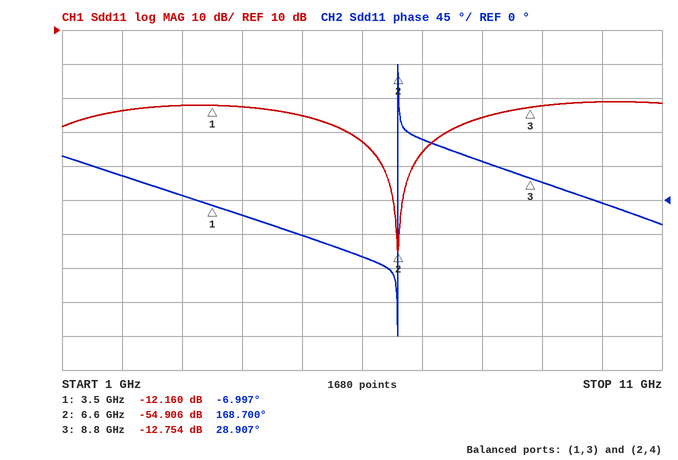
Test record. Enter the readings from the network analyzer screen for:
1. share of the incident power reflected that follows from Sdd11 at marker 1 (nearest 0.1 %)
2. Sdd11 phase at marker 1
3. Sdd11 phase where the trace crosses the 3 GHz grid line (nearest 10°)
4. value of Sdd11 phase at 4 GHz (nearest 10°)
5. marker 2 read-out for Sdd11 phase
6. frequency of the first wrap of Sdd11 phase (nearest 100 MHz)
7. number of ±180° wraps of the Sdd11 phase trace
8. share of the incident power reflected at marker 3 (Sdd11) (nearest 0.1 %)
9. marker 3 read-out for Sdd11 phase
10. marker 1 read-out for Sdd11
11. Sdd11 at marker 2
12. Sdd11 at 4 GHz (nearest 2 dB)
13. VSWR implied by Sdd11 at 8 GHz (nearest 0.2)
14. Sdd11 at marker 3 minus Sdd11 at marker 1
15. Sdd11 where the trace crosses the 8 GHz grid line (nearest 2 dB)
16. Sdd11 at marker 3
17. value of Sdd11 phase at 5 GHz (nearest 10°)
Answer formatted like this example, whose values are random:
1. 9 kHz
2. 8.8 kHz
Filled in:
1. 6.1 %
2. -6.997°
3. 10°
4. -20°
5. 168.700°
6. 6.6 GHz
7. 1
8. 5.3 %
9. 28.907°
10. -12.160 dB
11. -54.906 dB
12. -12 dB
13. 1.4
14. -0.594 dB
15. -16 dB
16. -12.754 dB
17. -50°
